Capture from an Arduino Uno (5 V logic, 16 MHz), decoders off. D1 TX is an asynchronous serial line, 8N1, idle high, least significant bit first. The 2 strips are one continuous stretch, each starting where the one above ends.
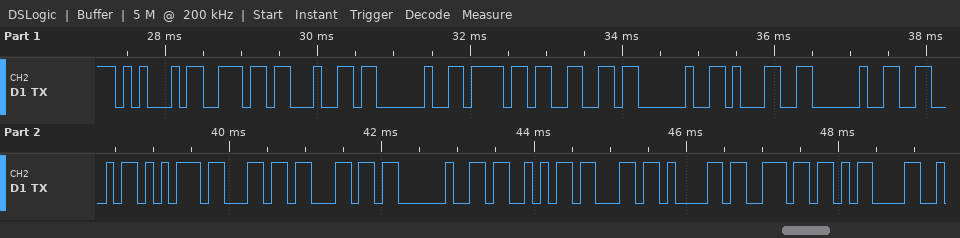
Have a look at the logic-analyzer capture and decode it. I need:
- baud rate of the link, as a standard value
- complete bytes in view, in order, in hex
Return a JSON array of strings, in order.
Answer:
["9600 baud", "0x45 0x6E 0x64 0x20 0x6F 0x66 0x20 0x31 0x20 0x46 0x75 0x6C 0x6C 0x20 0x53 0x63 0x61 0x6E 0x0D"]
